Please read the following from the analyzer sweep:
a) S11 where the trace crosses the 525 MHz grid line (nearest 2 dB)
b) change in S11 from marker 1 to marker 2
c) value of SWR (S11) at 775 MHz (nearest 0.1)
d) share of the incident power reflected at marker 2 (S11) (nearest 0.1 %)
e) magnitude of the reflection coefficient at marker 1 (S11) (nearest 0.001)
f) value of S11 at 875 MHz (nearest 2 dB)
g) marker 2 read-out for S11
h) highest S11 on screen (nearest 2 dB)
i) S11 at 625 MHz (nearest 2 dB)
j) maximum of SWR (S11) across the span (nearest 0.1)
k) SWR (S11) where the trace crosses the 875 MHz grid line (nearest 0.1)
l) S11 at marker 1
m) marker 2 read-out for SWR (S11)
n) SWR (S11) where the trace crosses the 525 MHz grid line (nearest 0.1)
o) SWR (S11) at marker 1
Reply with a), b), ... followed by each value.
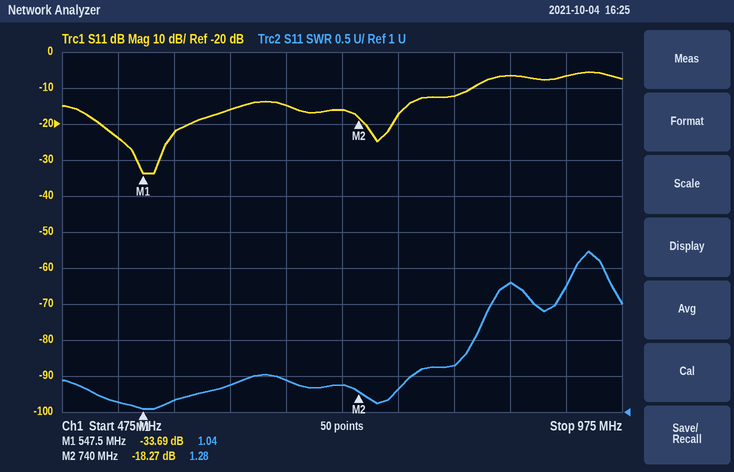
a) -24 dB
b) 15.42 dB
c) 1.3
d) 1.5 %
e) 0.021
f) -6 dB
g) -18.27 dB
h) -6 dB
i) -16 dB
j) 3.2
k) 2.8
l) -33.69 dB
m) 1.28
n) 1.1
o) 1.04
